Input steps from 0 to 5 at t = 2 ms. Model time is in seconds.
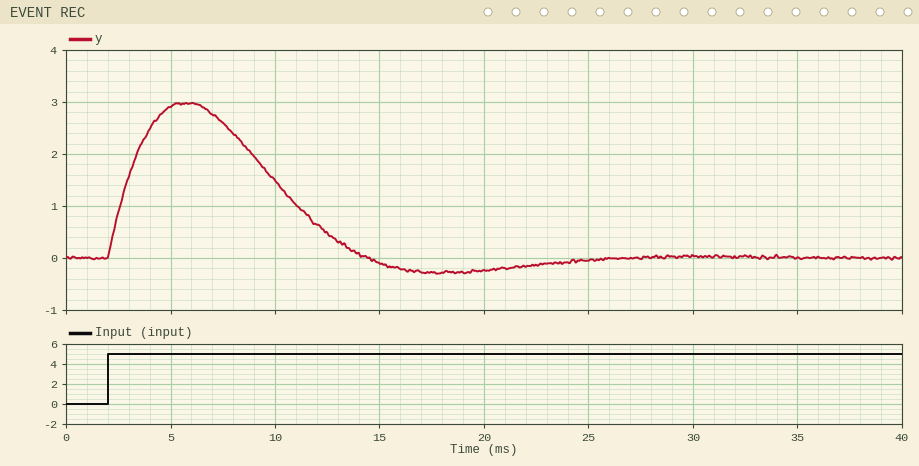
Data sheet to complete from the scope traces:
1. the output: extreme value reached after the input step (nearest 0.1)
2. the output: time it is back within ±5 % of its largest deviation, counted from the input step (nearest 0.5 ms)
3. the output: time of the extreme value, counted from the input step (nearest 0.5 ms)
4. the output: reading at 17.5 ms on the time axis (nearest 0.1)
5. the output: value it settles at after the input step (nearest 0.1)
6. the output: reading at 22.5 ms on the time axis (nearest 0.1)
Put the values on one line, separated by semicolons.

3.0; 20.0 ms; 3.5 ms; -0.3; 0.0; -0.1
